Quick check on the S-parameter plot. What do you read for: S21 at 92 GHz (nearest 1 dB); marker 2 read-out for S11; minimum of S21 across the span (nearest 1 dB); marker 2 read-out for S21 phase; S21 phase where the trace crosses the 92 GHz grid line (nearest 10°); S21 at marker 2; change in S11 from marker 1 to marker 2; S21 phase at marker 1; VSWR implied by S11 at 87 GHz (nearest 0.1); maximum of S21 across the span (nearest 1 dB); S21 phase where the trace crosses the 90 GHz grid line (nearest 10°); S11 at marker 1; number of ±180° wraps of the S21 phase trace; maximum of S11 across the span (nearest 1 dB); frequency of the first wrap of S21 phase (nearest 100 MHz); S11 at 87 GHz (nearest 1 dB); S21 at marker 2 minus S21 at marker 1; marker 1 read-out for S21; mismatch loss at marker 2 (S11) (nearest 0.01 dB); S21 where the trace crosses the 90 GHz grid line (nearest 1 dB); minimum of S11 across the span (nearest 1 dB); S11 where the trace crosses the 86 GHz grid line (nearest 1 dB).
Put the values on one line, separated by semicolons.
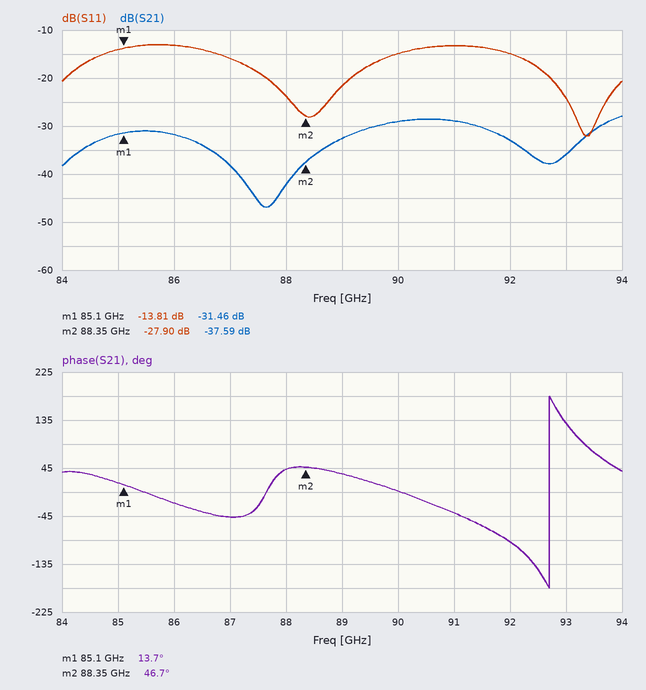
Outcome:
-33 dB; -27.90 dB; -47 dB; 46.7°; -90°; -37.59 dB; -14.09 dB; 13.7°; 1.4; -28 dB; 0°; -13.81 dB; 1; -13 dB; 92.7 GHz; -16 dB; -6.13 dB; -31.46 dB; 0.01 dB; -29 dB; -32 dB; -13 dB
